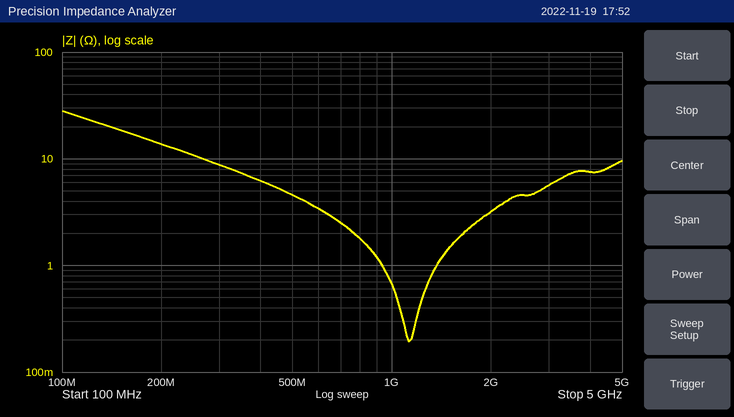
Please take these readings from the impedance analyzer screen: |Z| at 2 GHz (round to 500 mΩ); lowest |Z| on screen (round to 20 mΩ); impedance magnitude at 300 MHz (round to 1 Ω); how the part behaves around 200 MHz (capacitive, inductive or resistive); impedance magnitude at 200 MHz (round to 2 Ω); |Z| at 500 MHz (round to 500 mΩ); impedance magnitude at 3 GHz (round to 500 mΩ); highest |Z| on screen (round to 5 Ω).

3.0 Ω
200 mΩ
9 Ω
capacitive
14 Ω
4.5 Ω
5.5 Ω
30 Ω
